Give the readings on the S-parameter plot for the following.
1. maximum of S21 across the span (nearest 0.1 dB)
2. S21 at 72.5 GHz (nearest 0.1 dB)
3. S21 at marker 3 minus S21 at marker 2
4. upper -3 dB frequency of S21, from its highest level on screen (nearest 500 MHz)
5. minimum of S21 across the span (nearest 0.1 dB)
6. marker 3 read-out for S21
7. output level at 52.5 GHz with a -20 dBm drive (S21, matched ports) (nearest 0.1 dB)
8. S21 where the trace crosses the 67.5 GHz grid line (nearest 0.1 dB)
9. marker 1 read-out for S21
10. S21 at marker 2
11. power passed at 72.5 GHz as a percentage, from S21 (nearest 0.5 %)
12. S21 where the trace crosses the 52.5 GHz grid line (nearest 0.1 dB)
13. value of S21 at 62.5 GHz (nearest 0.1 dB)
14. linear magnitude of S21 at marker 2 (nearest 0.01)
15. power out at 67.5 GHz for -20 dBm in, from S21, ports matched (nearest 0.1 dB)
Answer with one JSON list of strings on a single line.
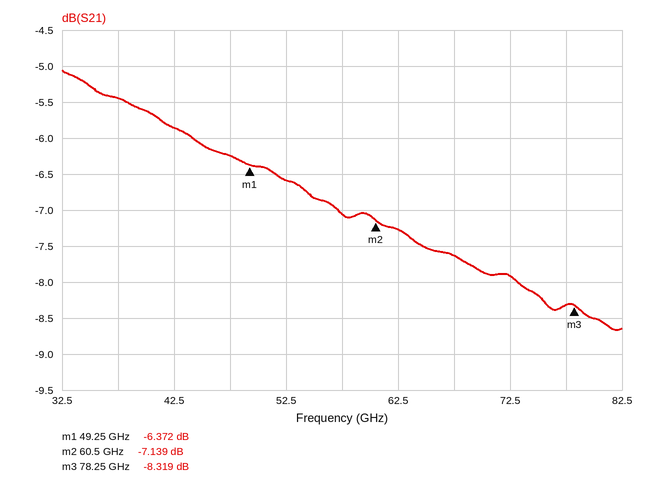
["-5.1 dB", "-7.9 dB", "-1.180 dB", "73.5 GHz", "-8.7 dB", "-8.319 dB", "-26.6 dBm", "-7.6 dB", "-6.372 dB", "-7.139 dB", "16.0 %", "-6.6 dB", "-7.3 dB", "0.44", "-27.6 dBm"]
